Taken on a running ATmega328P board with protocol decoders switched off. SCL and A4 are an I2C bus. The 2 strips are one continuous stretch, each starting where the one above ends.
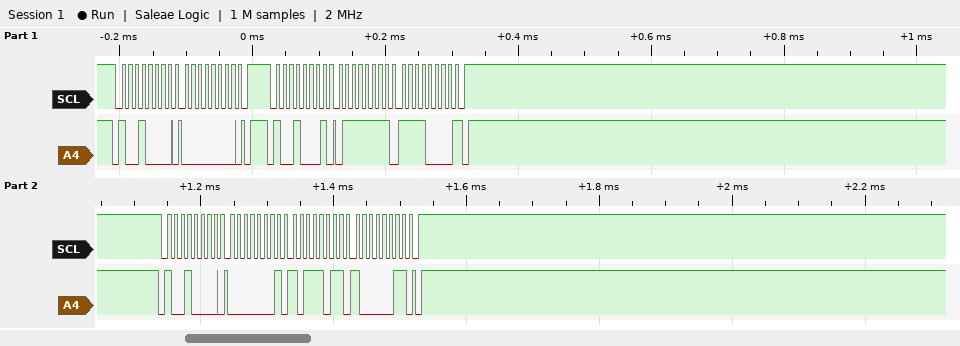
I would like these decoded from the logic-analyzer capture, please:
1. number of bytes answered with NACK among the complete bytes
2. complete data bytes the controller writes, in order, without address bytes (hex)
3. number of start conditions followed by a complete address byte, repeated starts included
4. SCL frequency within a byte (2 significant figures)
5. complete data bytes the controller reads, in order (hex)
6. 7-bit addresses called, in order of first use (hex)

1
00 01 BB 83
3
100 kHz
7F F0
0x48
